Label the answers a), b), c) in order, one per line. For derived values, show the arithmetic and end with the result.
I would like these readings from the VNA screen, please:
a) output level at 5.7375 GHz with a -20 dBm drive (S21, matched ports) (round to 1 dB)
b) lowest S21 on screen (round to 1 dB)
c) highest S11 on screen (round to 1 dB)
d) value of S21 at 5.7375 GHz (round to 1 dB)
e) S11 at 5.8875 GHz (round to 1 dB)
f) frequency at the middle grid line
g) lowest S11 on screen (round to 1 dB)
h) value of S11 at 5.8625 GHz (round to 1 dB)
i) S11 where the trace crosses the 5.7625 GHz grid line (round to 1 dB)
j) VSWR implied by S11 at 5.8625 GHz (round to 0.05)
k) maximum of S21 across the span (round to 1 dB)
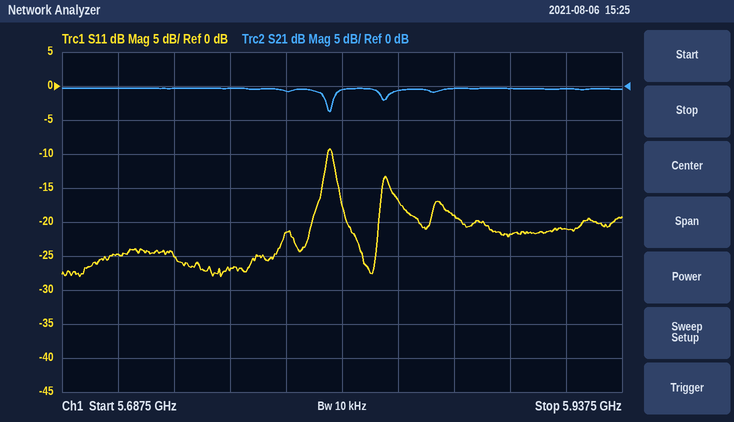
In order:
a) -20 dBm + (0 dB) = -20 dBm
b) -4 dB
c) -9 dB
d) 0 dB
e) -22 dB
f) 5.8125 GHz
g) -28 dB
h) -19 dB
i) -27 dB
j) |Γ| = 10^(-19/20) = 0.1122; VSWR = (1 + 0.1122)/(1 − 0.1122) ≈ 1.25
k) 0 dB
